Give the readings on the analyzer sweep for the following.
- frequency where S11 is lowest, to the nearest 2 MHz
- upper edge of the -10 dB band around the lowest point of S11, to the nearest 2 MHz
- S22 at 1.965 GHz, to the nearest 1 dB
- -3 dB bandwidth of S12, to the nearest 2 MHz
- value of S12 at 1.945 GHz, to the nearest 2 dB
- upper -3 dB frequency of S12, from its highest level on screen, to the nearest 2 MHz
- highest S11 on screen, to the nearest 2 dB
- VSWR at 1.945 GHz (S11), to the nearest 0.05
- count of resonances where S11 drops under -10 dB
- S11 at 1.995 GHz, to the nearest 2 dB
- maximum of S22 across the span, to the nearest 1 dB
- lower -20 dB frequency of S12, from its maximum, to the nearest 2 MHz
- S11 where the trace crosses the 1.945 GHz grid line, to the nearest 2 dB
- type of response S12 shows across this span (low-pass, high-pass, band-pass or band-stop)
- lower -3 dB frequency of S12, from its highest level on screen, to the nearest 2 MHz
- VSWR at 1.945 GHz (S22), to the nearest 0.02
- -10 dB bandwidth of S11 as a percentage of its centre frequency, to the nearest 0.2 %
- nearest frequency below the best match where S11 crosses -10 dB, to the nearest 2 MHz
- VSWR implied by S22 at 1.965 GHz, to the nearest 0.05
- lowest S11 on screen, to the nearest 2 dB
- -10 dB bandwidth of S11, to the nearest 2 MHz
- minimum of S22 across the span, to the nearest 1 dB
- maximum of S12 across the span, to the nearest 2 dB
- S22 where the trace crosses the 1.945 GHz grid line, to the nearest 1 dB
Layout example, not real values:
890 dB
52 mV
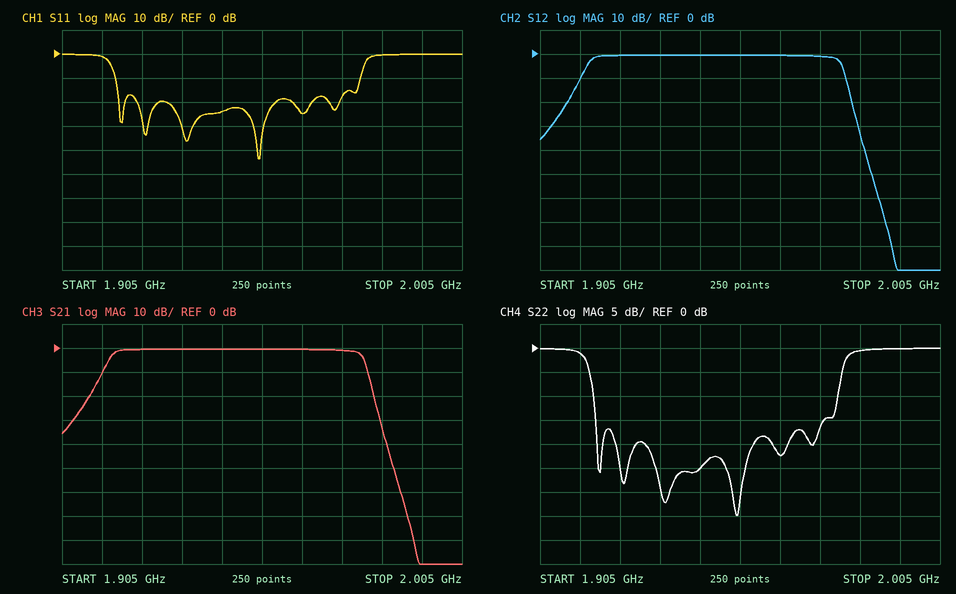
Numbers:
1.954 GHz
1.980 GHz
-22 dB
62 MHz
0 dB
1.980 GHz
0 dB
1.15
6
0 dB
0 dB
1.912 GHz
-24 dB
band-pass
1.918 GHz
1.12
3.2 %
1.918 GHz
1.15
-44 dB
62 MHz
-35 dB
0 dB
-25 dB
